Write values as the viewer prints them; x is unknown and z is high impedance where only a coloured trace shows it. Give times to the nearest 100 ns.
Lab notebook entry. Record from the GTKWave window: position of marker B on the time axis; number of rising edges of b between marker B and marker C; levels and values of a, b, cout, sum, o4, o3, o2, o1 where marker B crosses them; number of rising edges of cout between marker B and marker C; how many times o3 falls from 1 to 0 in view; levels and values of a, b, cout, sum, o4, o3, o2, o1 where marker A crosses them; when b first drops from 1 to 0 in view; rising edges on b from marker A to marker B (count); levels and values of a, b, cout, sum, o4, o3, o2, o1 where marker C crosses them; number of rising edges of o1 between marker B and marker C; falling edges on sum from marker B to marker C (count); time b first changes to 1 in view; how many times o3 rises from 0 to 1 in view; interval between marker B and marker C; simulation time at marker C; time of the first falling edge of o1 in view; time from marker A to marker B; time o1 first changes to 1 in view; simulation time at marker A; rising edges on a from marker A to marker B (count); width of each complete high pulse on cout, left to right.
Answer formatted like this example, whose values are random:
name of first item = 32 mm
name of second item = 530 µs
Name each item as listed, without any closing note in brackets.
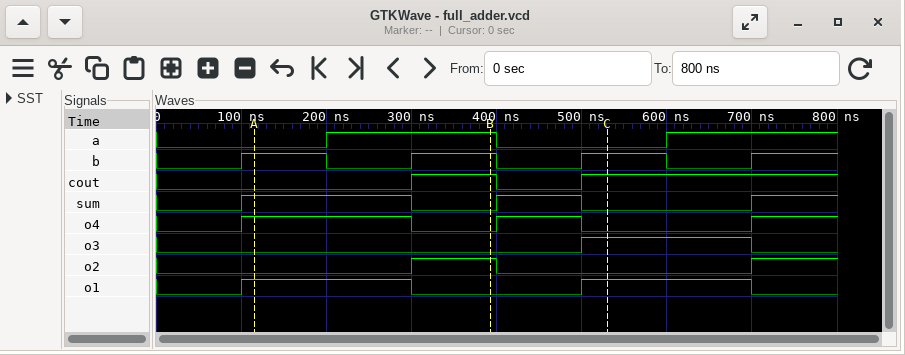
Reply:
position of marker B on the time axis = 400 ns
number of rising edges of b between marker B and marker C = 1
levels and values of a, b, cout, sum, o4, o3, o2, o1 where marker B crosses them = a=1, b=1, cout=1, sum=0, o4=0, o3=0, o2=1, o1=0
number of rising edges of cout between marker B and marker C = 1
how many times o3 falls from 1 to 0 in view = 1
levels and values of a, b, cout, sum, o4, o3, o2, o1 where marker A crosses them = a=0, b=1, cout=0, sum=1, o4=1, o3=0, o2=0, o1=1
when b first drops from 1 to 0 in view = 200 ns
rising edges on b from marker A to marker B = 1
levels and values of a, b, cout, sum, o4, o3, o2, o1 where marker C crosses them = a=0, b=1, cout=1, sum=0, o4=0, o3=1, o2=0, o1=1
number of rising edges of o1 between marker B and marker C = 1
falling edges on sum from marker B to marker C = 1
time b first changes to 1 in view = 100 ns
how many times o3 rises from 0 to 1 in view = 1
interval between marker B and marker C = 100 ns
simulation time at marker C = 500 ns
time of the first falling edge of o1 in view = 300 ns
time from marker A to marker B = 300 ns
time o1 first changes to 1 in view = 100 ns
simulation time at marker A = 100 ns
rising edges on a from marker A to marker B = 1
width of each complete high pulse on cout, left to right = 100 ns
